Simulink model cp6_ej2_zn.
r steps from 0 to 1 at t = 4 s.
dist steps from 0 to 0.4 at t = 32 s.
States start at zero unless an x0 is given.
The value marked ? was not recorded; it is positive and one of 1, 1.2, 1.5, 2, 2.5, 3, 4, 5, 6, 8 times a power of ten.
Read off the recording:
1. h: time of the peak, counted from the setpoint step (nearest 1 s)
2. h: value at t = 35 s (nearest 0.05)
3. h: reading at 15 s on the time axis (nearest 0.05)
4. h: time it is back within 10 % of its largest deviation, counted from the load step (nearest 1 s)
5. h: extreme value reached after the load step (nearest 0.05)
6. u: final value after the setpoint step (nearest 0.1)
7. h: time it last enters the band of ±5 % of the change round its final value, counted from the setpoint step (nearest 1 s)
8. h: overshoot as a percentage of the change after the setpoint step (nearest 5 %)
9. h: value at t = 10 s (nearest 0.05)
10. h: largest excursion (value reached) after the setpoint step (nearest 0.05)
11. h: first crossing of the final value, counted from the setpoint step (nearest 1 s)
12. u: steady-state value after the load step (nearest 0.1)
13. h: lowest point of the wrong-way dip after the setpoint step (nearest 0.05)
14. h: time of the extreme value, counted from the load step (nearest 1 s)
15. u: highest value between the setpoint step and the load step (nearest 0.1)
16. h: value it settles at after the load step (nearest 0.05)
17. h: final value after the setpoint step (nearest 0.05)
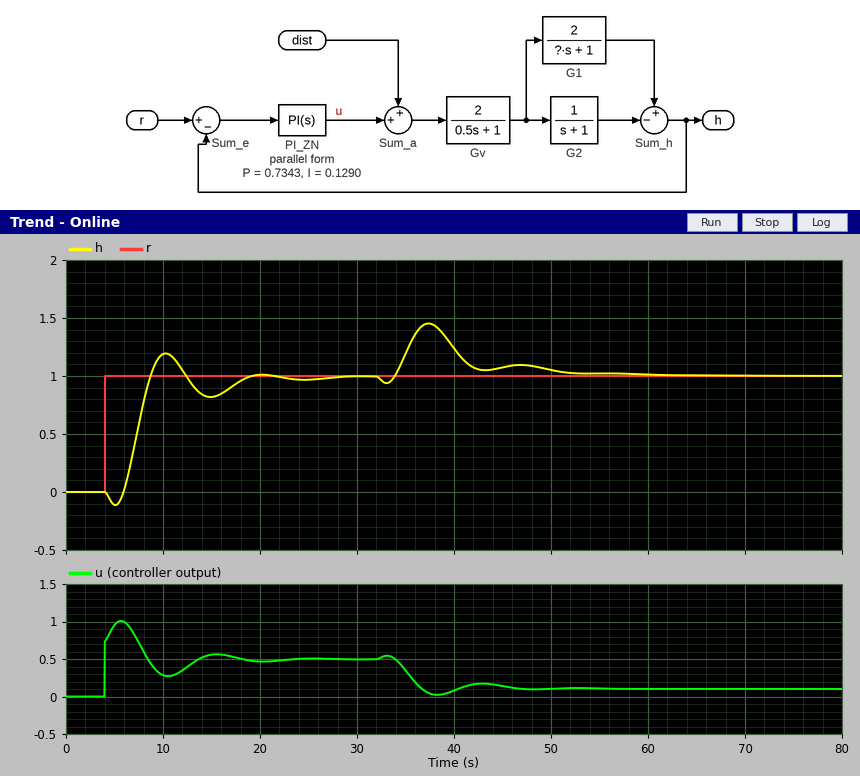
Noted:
6 s
1.20
0.80
18 s
1.45
0.5
14 s
20 %
1.20
1.20
5 s
0.1
-0.10
5 s
1.0
1.00
1.00
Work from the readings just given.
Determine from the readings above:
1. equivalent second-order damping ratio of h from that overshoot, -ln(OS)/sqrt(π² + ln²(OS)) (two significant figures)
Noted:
0.46
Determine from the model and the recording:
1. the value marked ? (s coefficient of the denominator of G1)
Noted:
3
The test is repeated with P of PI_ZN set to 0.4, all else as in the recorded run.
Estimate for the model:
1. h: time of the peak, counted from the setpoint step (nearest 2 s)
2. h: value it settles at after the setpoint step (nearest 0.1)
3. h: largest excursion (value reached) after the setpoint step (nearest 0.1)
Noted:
10 s
1.0
1.1
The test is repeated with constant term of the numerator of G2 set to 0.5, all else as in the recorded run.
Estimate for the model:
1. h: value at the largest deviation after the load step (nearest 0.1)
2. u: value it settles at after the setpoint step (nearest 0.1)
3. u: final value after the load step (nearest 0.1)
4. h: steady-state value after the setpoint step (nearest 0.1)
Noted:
1.4
0.3
-0.1
1.0
